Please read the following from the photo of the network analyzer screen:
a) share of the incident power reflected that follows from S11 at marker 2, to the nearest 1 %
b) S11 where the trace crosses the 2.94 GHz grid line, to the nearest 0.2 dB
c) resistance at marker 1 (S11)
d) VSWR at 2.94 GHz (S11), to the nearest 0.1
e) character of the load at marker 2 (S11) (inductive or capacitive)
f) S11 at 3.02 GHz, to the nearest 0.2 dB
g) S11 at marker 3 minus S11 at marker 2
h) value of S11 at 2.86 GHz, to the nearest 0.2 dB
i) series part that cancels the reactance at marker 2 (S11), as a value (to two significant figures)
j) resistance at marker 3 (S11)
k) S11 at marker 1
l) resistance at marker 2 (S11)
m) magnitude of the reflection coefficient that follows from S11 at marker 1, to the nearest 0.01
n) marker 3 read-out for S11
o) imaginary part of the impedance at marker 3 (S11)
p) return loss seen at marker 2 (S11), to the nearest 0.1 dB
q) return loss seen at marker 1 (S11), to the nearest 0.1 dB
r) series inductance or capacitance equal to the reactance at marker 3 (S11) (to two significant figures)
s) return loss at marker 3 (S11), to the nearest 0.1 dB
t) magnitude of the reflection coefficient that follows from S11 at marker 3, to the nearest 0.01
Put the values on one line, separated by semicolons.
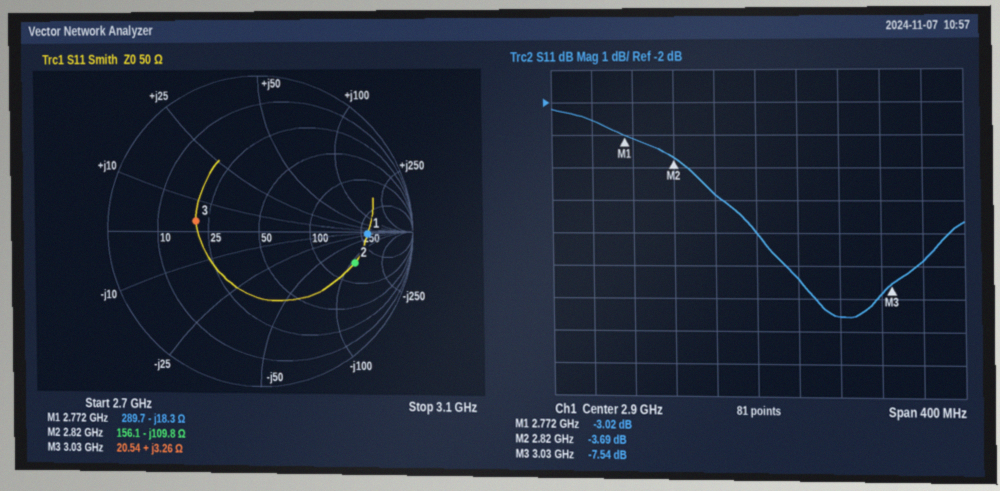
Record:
43 %; -7.4 dB; 289.7 Ω; 2.5; capacitive; -7.8 dB; -3.85 dB; -4.8 dB; 6.2 nH; 20.54 Ω; -3.02 dB; 156.1 Ω; 0.71; -7.54 dB; +3.26 Ω; 3.7 dB; 3.0 dB; 170 pH; 7.5 dB; 0.42
